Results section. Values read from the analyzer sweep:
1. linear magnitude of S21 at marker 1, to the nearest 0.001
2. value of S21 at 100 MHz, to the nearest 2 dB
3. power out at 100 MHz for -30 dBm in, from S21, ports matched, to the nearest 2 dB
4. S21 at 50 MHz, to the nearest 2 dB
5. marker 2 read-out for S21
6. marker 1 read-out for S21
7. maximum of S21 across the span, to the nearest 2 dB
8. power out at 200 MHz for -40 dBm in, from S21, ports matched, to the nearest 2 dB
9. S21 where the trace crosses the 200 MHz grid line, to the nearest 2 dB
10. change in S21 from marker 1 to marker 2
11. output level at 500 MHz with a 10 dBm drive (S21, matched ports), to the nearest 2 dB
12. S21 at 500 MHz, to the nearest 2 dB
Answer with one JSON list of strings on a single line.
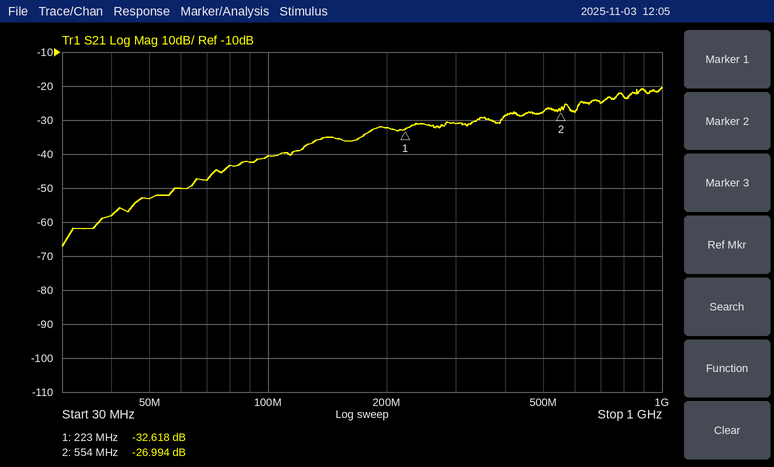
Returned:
["0.023", "-40 dB", "-70 dBm", "-54 dB", "-26.994 dB", "-32.618 dB", "-20 dB", "-72 dBm", "-32 dB", "5.624 dB", "-18 dBm", "-28 dB"]
